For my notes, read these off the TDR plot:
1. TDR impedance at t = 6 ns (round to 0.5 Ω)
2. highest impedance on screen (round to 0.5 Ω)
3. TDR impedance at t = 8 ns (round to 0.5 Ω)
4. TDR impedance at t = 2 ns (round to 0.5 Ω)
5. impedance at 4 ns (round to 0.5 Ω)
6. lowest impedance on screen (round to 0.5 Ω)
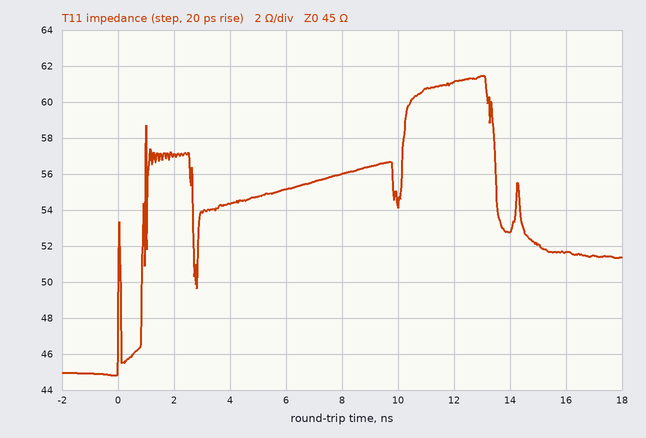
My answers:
55.0 Ω
61.5 Ω
56.0 Ω
57.0 Ω
54.5 Ω
45.0 Ω
